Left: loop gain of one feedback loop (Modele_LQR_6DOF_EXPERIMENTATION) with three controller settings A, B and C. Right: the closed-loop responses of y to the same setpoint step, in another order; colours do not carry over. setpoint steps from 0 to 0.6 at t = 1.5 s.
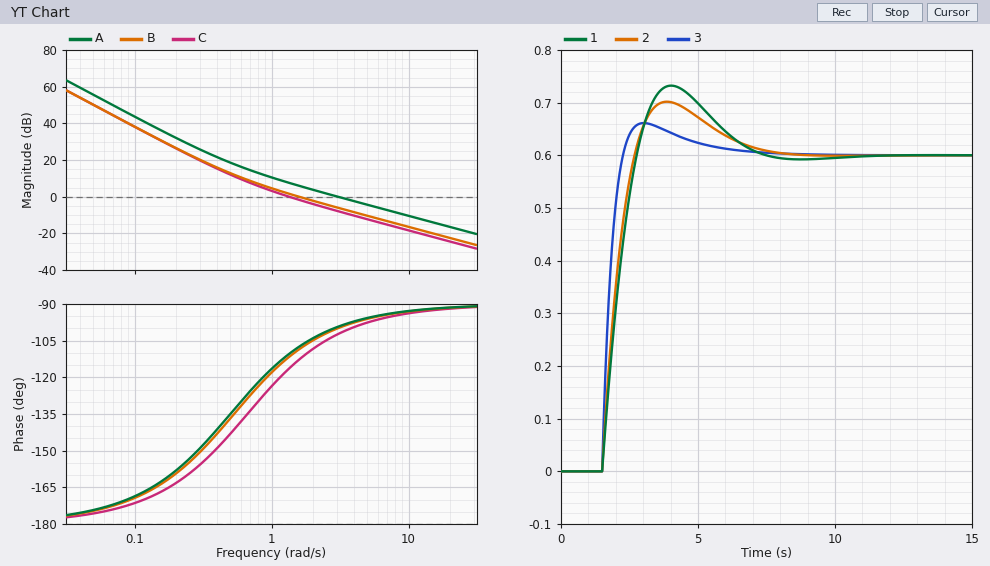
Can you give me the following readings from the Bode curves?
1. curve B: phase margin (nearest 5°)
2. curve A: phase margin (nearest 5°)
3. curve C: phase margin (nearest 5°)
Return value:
70°
80°
65°
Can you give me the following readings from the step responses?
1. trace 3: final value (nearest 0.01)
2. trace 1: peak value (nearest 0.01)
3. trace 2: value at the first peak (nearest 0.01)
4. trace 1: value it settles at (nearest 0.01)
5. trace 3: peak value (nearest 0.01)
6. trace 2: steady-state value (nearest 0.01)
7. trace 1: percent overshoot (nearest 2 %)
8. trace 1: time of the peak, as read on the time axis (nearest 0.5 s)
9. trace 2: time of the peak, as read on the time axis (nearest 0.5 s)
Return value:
0.60
0.73
0.70
0.60
0.66
0.60
22 %
4.0 s
4.0 s
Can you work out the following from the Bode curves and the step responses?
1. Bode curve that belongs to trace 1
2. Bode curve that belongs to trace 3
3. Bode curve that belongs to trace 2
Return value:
C
A
B
